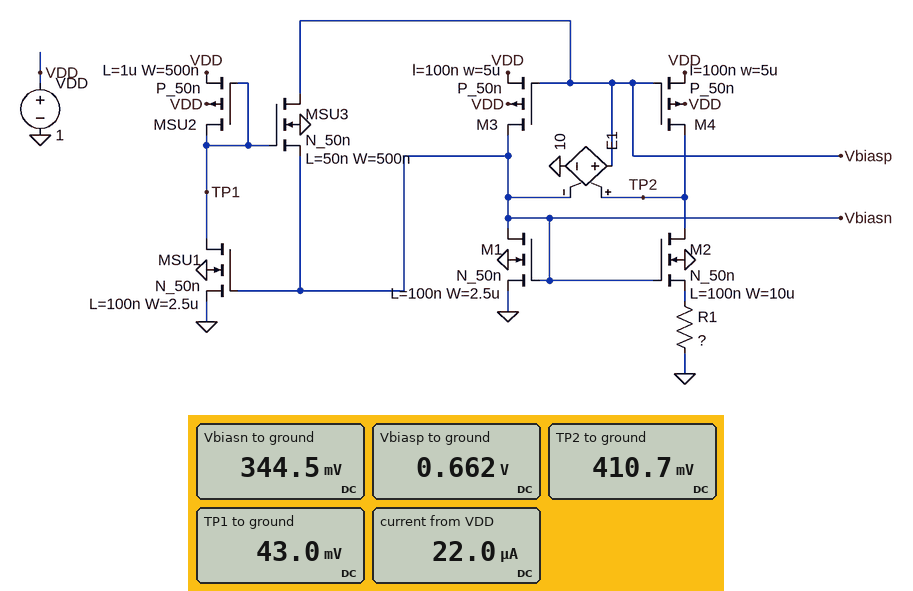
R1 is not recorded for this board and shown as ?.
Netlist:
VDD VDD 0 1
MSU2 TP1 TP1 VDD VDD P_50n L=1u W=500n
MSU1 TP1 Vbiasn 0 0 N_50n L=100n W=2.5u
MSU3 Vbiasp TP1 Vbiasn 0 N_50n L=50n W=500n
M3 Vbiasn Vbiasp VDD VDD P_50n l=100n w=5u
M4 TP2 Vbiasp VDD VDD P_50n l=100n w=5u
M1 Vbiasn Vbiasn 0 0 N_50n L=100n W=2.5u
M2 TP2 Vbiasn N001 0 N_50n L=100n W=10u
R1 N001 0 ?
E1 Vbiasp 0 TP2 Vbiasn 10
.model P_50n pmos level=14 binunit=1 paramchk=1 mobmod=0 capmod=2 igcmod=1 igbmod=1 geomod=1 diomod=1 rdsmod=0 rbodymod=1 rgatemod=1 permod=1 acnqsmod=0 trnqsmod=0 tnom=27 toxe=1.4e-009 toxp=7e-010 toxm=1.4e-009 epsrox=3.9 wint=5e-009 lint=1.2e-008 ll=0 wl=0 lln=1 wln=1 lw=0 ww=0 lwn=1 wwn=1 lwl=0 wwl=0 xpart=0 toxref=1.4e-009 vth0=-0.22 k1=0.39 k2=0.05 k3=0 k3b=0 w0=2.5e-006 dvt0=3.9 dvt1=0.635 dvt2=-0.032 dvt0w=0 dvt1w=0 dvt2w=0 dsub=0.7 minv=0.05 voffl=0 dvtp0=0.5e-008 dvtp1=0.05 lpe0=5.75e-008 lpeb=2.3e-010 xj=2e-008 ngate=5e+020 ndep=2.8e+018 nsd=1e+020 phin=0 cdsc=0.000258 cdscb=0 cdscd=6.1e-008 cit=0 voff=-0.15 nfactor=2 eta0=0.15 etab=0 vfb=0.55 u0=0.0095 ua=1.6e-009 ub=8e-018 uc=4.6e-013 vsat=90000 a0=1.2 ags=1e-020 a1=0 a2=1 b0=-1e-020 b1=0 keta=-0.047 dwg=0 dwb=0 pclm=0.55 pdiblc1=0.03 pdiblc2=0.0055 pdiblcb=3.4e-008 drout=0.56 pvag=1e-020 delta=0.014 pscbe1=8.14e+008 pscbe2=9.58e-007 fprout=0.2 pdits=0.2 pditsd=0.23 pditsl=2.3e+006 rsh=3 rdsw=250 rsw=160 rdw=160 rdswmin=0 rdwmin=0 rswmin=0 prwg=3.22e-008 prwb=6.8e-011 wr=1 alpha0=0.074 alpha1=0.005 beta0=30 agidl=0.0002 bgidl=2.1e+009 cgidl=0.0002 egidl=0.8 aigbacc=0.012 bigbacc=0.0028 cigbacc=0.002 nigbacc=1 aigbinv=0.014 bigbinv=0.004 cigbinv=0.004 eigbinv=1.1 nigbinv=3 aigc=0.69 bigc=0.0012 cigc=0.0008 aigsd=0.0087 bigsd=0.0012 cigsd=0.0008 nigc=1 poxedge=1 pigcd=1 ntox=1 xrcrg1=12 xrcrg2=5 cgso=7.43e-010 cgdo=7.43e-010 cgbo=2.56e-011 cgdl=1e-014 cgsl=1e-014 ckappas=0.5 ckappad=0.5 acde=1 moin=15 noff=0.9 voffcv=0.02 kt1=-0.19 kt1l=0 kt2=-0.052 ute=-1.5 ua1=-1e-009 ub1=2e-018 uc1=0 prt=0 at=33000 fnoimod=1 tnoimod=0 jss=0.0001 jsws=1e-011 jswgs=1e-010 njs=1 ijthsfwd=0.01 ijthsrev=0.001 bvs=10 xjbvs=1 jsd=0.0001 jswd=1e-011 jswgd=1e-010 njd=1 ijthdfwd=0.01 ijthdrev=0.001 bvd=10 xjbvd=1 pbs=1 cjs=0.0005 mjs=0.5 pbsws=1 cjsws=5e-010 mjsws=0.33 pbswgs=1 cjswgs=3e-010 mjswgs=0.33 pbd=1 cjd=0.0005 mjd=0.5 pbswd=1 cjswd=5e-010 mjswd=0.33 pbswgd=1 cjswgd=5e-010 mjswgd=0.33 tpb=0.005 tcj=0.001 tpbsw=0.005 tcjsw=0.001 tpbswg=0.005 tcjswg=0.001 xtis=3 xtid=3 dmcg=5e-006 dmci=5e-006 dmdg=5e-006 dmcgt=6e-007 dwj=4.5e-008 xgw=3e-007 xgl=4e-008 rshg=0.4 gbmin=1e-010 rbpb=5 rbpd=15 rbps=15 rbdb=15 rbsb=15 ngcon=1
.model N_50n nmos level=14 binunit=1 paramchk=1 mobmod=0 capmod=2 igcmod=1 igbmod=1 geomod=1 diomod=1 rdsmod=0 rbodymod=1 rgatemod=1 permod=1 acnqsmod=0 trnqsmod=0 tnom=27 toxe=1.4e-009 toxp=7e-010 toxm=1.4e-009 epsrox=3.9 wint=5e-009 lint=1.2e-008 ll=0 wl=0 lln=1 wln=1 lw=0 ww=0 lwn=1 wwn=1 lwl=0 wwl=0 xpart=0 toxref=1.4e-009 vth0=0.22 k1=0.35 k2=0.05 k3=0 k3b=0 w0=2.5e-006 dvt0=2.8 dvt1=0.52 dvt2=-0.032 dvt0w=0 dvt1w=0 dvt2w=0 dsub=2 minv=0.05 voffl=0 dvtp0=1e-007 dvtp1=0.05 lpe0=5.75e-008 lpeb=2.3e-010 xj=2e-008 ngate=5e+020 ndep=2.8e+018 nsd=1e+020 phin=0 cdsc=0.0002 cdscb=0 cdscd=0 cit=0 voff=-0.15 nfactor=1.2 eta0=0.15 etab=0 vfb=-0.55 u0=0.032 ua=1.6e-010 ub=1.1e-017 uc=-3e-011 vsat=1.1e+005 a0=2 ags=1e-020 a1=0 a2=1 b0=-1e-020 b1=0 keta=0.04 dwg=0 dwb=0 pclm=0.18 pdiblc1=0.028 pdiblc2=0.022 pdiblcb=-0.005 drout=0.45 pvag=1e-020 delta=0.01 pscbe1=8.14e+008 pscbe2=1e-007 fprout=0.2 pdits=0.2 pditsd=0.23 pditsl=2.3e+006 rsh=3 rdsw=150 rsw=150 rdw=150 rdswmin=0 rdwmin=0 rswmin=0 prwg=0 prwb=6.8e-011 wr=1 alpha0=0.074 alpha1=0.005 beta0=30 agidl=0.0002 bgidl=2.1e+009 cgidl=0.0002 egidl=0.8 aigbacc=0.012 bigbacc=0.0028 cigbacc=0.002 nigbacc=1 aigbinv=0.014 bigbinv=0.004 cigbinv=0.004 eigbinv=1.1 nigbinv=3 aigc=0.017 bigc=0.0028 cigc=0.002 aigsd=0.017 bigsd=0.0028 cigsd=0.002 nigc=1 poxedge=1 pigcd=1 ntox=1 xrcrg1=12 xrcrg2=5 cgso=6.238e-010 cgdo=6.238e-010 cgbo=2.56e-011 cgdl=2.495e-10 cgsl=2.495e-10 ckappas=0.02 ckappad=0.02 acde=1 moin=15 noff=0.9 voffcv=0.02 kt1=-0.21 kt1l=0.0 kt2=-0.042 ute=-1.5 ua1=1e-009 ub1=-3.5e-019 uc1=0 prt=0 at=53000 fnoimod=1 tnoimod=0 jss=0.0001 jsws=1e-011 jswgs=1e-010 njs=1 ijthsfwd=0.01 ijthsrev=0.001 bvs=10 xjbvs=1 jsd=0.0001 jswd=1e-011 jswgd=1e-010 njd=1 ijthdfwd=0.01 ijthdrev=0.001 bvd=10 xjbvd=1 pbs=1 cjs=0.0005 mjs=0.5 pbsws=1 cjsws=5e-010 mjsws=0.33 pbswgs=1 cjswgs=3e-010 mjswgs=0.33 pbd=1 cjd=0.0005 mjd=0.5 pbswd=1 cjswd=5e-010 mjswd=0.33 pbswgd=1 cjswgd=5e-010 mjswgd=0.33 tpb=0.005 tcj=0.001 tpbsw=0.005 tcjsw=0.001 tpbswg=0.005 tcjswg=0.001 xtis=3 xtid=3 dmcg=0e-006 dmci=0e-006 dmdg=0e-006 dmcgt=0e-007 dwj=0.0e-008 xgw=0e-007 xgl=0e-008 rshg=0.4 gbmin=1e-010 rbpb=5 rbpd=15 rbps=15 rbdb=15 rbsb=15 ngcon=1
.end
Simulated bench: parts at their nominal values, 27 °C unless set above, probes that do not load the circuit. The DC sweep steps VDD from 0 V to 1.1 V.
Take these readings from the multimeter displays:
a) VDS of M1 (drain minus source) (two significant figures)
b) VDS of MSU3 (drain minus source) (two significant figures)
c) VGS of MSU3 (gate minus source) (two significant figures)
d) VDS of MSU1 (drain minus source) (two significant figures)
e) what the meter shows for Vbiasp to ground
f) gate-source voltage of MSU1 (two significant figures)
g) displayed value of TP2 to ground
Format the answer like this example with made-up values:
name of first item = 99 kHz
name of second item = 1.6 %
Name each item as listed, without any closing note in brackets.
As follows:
VDS of M1 (drain minus source) = 340 mV
VDS of MSU3 (drain minus source) = 320 mV
VGS of MSU3 (gate minus source) = -300 mV
VDS of MSU1 (drain minus source) = 43 mV
what the meter shows for Vbiasp to ground = 0.662 V
gate-source voltage of MSU1 = 340 mV
displayed value of TP2 to ground = 410.7 mV
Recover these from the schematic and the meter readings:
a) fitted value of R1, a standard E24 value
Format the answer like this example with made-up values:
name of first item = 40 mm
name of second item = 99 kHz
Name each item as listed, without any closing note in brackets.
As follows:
fitted value of R1, a standard E24 value = 6.8 kΩ
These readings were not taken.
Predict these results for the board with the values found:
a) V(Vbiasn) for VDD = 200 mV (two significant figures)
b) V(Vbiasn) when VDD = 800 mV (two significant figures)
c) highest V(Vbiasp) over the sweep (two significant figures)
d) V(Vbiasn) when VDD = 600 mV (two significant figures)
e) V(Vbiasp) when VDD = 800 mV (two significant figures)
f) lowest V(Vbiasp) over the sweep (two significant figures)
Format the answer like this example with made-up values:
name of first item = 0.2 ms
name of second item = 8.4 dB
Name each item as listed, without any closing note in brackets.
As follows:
V(Vbiasn) for VDD = 200 mV = 200 mV
V(Vbiasn) when VDD = 800 mV = 340 mV
highest V(Vbiasp) over the sweep = 760 mV
V(Vbiasn) when VDD = 600 mV = 340 mV
V(Vbiasp) when VDD = 800 mV = 460 mV
lowest V(Vbiasp) over the sweep = -96 mV
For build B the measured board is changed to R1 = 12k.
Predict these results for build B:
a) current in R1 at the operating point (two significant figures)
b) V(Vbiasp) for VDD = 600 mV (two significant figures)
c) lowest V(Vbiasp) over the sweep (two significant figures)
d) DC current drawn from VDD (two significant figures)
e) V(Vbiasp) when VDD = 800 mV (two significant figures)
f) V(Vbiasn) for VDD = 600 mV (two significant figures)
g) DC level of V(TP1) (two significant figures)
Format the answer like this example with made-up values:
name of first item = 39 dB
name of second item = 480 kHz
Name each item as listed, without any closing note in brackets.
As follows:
current in R1 at the operating point = 4.4 µA
V(Vbiasp) for VDD = 600 mV = 290 mV
lowest V(Vbiasp) over the sweep = -87 mV
DC current drawn from VDD = 13 µA
V(Vbiasp) when VDD = 800 mV = 490 mV
V(Vbiasn) for VDD = 600 mV = 310 mV
DC level of V(TP1) = 190 mV
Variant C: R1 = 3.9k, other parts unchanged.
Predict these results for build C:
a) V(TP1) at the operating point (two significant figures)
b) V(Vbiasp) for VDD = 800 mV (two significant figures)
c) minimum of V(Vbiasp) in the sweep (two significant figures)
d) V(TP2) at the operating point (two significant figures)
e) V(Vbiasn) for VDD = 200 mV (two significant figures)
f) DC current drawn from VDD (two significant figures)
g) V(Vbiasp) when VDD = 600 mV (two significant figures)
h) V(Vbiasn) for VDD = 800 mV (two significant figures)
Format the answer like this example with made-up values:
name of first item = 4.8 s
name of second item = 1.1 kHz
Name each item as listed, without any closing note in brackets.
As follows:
V(TP1) at the operating point = 21 mV
V(Vbiasp) for VDD = 800 mV = 420 mV
minimum of V(Vbiasp) in the sweep = -110 mV
V(TP2) at the operating point = 440 mV
V(Vbiasn) for VDD = 200 mV = 200 mV
DC current drawn from VDD = 37 µA
V(Vbiasp) when VDD = 600 mV = 220 mV
V(Vbiasn) for VDD = 800 mV = 380 mV
